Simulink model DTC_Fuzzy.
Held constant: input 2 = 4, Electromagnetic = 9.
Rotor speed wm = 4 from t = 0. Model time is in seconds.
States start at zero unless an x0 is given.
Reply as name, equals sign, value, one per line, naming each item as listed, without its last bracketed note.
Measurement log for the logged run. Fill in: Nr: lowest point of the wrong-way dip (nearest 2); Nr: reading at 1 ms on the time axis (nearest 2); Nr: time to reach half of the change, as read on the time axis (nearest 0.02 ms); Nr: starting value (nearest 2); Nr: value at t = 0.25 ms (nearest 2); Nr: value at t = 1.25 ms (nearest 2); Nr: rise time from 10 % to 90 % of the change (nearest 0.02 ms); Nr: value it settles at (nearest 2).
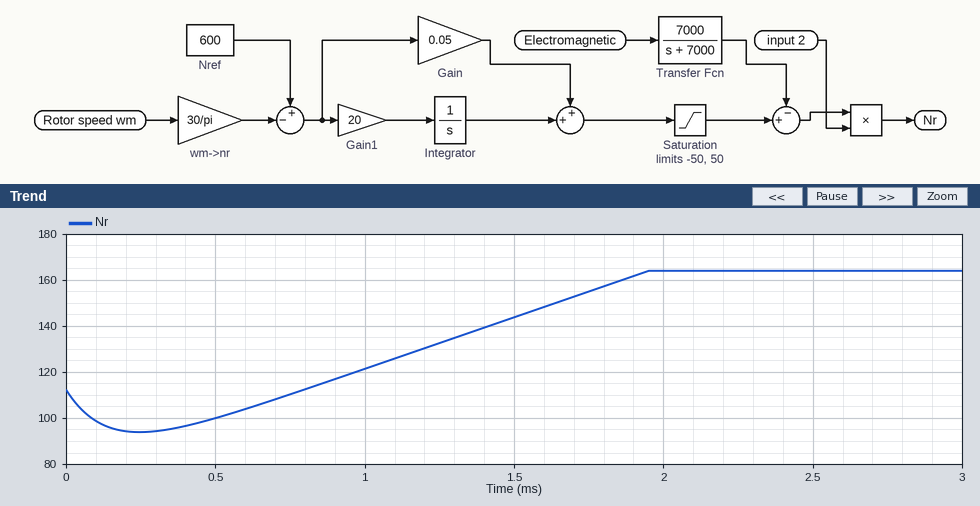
Nr: lowest point of the wrong-way dip = 94
Nr: reading at 1 ms on the time axis = 122
Nr: time to reach half of the change, as read on the time axis = 1.38 ms
Nr: starting value = 112
Nr: value at t = 0.25 ms = 94
Nr: value at t = 1.25 ms = 132
Nr: rise time from 10 % to 90 % of the change = 0.92 ms
Nr: value it settles at = 164
